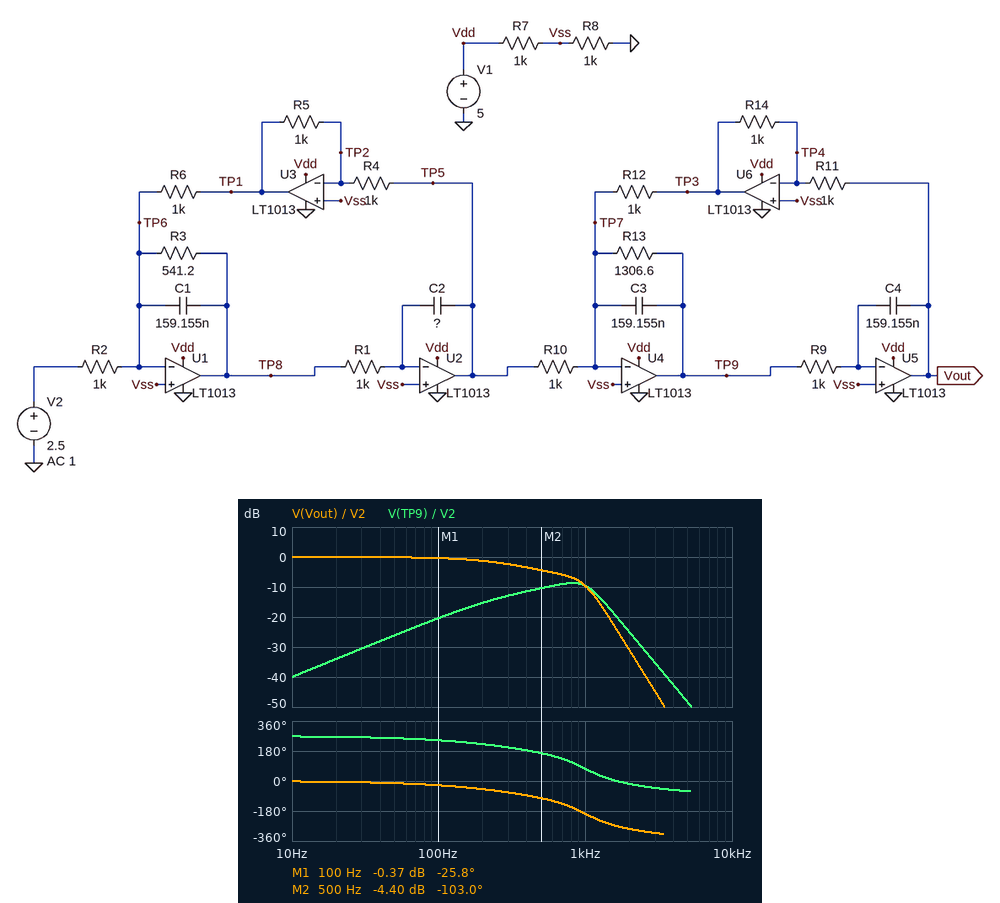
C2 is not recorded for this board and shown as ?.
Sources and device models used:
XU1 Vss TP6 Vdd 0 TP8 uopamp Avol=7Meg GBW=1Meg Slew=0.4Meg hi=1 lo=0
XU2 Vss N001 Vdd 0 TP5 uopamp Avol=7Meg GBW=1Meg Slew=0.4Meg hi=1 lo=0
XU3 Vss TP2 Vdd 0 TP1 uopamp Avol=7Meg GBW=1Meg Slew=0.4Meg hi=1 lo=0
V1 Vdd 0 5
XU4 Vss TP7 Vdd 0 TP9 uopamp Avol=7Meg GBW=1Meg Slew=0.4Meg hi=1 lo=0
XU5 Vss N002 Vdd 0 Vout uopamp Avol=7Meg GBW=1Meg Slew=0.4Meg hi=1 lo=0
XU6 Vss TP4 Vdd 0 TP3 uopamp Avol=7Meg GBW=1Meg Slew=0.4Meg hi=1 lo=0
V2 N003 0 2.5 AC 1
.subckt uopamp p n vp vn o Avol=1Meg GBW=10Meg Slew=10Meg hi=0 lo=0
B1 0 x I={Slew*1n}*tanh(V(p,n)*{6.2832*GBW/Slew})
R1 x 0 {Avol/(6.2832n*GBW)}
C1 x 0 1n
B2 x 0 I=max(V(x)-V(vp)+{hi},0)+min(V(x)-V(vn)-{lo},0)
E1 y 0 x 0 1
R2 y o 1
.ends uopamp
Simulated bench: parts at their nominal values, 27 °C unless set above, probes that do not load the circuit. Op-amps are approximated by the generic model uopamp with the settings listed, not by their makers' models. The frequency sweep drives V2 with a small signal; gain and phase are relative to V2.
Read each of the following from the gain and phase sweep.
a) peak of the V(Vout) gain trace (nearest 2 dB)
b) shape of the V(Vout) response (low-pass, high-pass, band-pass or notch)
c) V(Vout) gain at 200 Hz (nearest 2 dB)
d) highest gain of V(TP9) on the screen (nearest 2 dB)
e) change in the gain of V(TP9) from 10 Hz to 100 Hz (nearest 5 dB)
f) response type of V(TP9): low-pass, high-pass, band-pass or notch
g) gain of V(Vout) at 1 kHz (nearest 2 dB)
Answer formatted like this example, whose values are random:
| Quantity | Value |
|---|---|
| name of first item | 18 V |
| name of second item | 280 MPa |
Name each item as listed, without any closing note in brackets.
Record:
| Quantity | Value |
|---|---|
| peak of the V(Vout) gain trace | 0 dB |
| shape of the V(Vout) response | low-pass |
| V(Vout) gain at 200 Hz | -2 dB |
| highest gain of V(TP9) on the screen | -8 dB |
| change in the gain of V(TP9) from 10 Hz to 100 Hz | 20 dB |
| response type of V(TP9): low-pass, high-pass, band-pass or notch | band-pass |
| gain of V(Vout) at 1 kHz | -10 dB |
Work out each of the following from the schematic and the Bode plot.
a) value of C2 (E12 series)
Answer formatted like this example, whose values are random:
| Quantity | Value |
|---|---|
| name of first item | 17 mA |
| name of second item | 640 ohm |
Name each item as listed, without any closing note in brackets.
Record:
| Quantity | Value |
|---|---|
| value of C2 | 330 nF |
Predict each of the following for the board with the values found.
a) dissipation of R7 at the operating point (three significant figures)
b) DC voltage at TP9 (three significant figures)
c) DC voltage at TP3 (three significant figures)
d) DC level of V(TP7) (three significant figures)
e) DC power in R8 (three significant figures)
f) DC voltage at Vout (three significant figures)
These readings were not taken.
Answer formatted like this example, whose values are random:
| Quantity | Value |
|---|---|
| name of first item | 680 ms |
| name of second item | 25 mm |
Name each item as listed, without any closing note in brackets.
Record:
| Quantity | Value |
|---|---|
| dissipation of R7 at the operating point | 6.25 mW |
| DC voltage at TP9 | 2.50 V |
| DC voltage at TP3 | 2.50 V |
| DC level of V(TP7) | 2.50 V |
| DC power in R8 | 6.25 mW |
| DC voltage at Vout | 2.50 V |
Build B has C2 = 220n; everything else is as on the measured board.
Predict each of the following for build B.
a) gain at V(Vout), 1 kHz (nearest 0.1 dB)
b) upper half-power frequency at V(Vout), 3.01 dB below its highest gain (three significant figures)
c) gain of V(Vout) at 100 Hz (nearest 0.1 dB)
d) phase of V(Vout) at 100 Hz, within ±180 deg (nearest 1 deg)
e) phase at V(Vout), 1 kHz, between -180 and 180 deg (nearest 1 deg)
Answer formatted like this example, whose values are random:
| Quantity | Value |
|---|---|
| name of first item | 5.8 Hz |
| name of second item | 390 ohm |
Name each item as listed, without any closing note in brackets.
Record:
| Quantity | Value |
|---|---|
| gain at V(Vout), 1 kHz | -5.9 dB |
| upper half-power frequency at V(Vout), 3.01 dB below its highest gain | 776 Hz |
| gain of V(Vout) at 100 Hz | -0.1 dB |
| phase of V(Vout) at 100 Hz, within ±180 deg | -19 deg |
| phase at V(Vout), 1 kHz, between -180 and 180 deg | 171 deg |
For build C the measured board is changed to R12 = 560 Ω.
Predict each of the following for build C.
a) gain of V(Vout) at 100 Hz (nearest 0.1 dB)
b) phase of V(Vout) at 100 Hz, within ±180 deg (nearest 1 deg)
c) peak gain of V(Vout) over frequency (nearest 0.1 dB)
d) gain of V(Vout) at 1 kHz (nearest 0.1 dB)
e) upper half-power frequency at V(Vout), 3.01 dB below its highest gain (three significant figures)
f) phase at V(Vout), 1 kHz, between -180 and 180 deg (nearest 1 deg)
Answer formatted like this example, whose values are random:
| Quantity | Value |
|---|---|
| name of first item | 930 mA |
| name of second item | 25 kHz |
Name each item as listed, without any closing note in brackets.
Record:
| Quantity | Value |
|---|---|
| gain of V(Vout) at 100 Hz | -5.4 dB |
| phase of V(Vout) at 100 Hz, within ±180 deg | -24 deg |
| peak gain of V(Vout) over frequency | -5.0 dB |
| gain of V(Vout) at 1 kHz | -12.7 dB |
| upper half-power frequency at V(Vout), 3.01 dB below its highest gain | 334 Hz |
| phase at V(Vout), 1 kHz, between -180 and 180 deg | -150 deg |
